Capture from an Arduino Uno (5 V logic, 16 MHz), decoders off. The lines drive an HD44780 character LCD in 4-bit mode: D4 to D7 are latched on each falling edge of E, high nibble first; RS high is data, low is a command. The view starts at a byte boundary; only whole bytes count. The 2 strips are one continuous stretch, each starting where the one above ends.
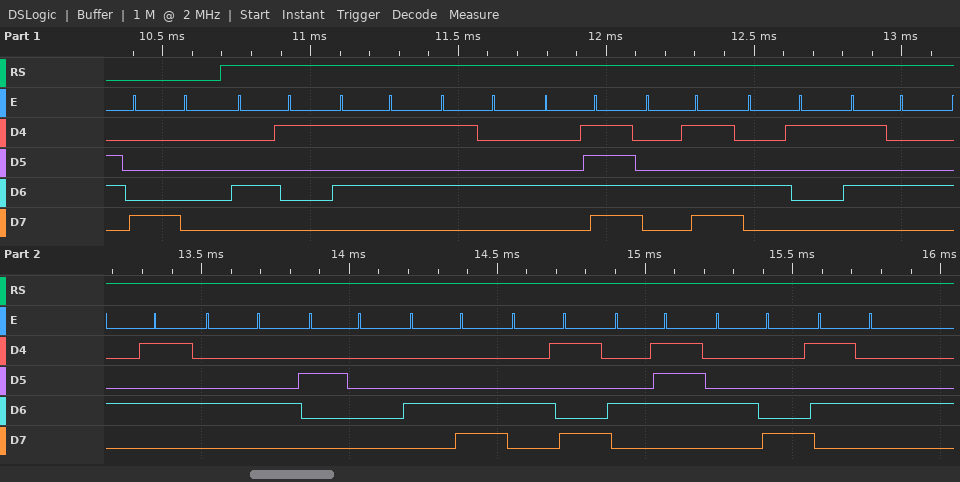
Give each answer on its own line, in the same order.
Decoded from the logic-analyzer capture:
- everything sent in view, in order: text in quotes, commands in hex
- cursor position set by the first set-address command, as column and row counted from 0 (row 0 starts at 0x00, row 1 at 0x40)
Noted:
0x80 "AUTOMATED LIGHT"
column 0, row 0
